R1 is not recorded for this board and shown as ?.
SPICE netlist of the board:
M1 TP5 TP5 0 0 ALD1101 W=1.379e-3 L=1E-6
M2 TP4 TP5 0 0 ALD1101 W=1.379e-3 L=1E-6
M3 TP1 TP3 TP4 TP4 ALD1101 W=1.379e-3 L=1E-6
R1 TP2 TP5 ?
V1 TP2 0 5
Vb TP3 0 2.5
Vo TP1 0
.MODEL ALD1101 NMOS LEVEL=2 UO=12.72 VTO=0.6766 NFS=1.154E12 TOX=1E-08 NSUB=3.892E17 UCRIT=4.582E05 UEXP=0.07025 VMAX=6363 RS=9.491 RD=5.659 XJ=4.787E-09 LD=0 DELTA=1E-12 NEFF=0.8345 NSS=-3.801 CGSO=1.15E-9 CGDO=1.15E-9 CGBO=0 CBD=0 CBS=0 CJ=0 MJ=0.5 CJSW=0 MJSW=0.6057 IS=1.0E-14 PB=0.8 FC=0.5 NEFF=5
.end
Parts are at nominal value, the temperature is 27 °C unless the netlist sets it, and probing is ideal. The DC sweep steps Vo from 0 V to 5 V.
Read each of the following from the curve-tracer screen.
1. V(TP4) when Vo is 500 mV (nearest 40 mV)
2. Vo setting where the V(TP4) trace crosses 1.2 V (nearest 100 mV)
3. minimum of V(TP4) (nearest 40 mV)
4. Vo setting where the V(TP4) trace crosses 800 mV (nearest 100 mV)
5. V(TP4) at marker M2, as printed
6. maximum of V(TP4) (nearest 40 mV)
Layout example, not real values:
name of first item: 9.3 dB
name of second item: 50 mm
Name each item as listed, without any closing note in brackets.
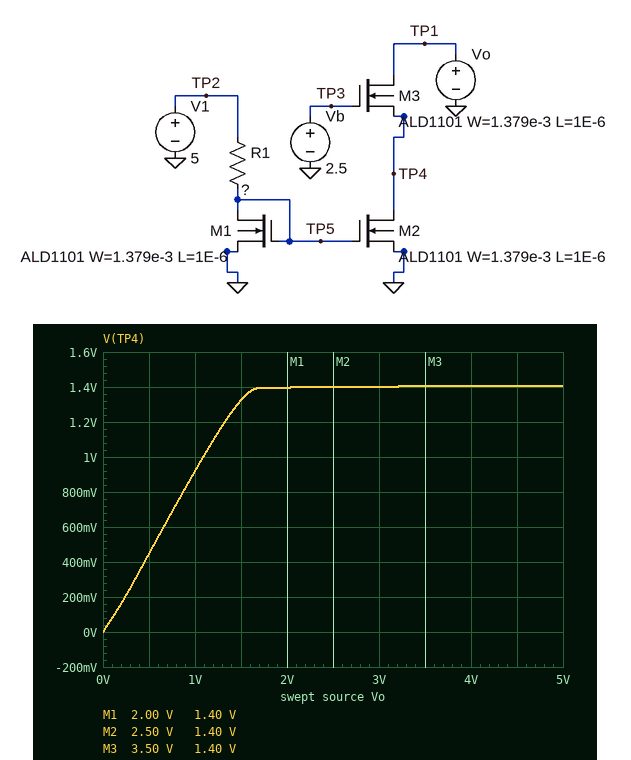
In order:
V(TP4) when Vo is 500 mV: 440 mV
Vo setting where the V(TP4) trace crosses 1.2 V: 1.3 V
minimum of V(TP4): 0 V
Vo setting where the V(TP4) trace crosses 800 mV: 900 mV
V(TP4) at marker M2, as printed: 1.40 V
maximum of V(TP4): 1.40 V
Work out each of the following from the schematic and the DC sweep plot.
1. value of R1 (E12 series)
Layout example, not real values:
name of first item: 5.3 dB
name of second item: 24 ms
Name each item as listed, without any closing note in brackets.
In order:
value of R1: 10 kΩ
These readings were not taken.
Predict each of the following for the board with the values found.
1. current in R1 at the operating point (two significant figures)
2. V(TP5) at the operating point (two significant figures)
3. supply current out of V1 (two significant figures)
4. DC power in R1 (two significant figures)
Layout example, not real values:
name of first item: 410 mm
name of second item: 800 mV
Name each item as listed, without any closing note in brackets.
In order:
current in R1 at the operating point: 390 µA
V(TP5) at the operating point: 1.1 V
supply current out of V1: 390 µA
DC power in R1: 1.5 mW
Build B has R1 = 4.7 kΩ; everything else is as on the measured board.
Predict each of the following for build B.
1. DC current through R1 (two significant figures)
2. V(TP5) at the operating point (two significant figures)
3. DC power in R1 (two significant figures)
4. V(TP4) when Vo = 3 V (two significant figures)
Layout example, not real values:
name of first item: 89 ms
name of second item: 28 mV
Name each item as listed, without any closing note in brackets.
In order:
DC current through R1: 790 µA
V(TP5) at the operating point: 1.3 V
DC power in R1: 2.9 mW
V(TP4) when Vo = 3 V: 1.2 V
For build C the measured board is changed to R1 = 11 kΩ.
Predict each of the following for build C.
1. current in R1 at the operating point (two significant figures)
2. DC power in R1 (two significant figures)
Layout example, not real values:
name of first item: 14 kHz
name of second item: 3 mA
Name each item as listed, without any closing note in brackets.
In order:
current in R1 at the operating point: 360 µA
DC power in R1: 1.4 mW
